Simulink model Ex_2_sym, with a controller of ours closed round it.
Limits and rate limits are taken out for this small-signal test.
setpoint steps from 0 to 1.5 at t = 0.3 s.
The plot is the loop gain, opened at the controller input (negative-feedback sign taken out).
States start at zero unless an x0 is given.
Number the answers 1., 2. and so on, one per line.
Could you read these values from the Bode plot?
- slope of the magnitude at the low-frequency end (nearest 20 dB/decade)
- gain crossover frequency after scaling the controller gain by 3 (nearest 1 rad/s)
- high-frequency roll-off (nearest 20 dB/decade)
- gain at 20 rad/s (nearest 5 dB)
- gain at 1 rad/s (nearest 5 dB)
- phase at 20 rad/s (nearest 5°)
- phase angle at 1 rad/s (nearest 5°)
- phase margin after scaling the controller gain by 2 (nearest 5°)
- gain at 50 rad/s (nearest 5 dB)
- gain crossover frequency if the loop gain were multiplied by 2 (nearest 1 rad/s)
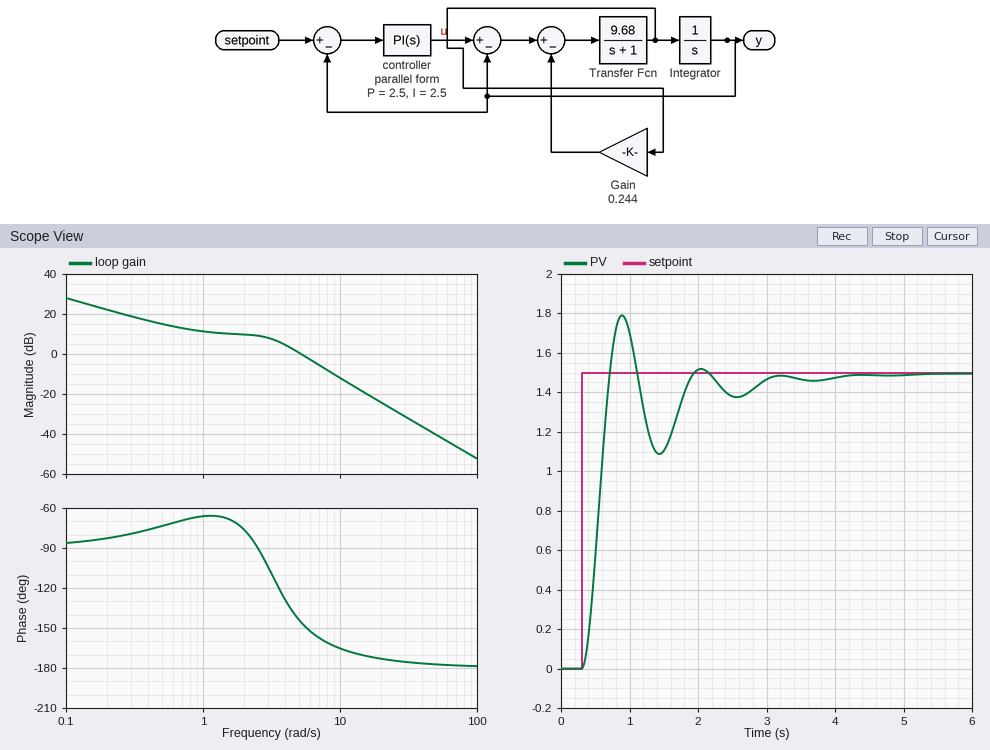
1. -20 dB/decade
2. 9 rad/s
3. -40 dB/decade
4. -25 dB
5. 10 dB
6. -175°
7. -65°
8. 20°
9. -40 dB
10. 7 rad/s
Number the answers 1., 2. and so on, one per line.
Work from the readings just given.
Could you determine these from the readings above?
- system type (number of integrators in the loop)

1. 1
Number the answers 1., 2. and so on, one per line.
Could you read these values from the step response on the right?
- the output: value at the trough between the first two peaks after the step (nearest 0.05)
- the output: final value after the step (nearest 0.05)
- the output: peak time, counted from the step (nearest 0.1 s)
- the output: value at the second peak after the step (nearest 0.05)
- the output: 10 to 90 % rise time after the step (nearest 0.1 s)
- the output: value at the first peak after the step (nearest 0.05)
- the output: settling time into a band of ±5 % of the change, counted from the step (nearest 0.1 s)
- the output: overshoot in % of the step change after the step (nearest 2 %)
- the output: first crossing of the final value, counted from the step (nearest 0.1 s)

1. 1.10
2. 1.50
3. 0.6 s
4. 1.50
5. 0.3 s
6. 1.80
7. 2.5 s
8. 20 %
9. 0.4 s
